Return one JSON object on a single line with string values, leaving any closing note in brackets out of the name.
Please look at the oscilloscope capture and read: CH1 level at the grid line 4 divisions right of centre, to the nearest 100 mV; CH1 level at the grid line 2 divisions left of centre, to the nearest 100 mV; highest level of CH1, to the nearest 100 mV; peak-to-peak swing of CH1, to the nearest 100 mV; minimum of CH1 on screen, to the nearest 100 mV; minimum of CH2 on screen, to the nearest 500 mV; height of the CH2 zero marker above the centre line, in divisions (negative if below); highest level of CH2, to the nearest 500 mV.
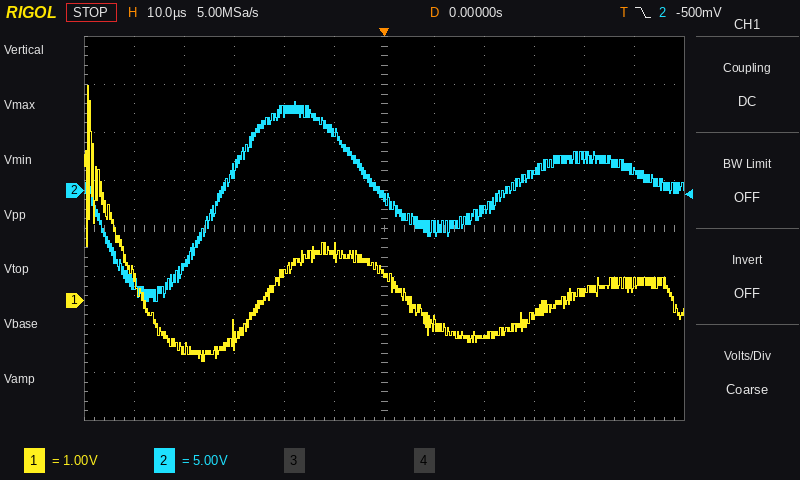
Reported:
{"CH1 level at the grid line 4 divisions right of centre, to the nearest 100 mV": "200 mV", "CH1 level at the grid line 2 divisions left of centre, to the nearest 100 mV": "600 mV", "highest level of CH1, to the nearest 100 mV": "4.5 V", "peak-to-peak swing of CH1, to the nearest 100 mV": "5.8 V", "minimum of CH1 on screen, to the nearest 100 mV": "-1.3 V", "minimum of CH2 on screen, to the nearest 500 mV": "-11.5 V", "height of the CH2 zero marker above the centre line, in divisions": "+0.8 div", "highest level of CH2, to the nearest 500 mV": "9.0 V"}
